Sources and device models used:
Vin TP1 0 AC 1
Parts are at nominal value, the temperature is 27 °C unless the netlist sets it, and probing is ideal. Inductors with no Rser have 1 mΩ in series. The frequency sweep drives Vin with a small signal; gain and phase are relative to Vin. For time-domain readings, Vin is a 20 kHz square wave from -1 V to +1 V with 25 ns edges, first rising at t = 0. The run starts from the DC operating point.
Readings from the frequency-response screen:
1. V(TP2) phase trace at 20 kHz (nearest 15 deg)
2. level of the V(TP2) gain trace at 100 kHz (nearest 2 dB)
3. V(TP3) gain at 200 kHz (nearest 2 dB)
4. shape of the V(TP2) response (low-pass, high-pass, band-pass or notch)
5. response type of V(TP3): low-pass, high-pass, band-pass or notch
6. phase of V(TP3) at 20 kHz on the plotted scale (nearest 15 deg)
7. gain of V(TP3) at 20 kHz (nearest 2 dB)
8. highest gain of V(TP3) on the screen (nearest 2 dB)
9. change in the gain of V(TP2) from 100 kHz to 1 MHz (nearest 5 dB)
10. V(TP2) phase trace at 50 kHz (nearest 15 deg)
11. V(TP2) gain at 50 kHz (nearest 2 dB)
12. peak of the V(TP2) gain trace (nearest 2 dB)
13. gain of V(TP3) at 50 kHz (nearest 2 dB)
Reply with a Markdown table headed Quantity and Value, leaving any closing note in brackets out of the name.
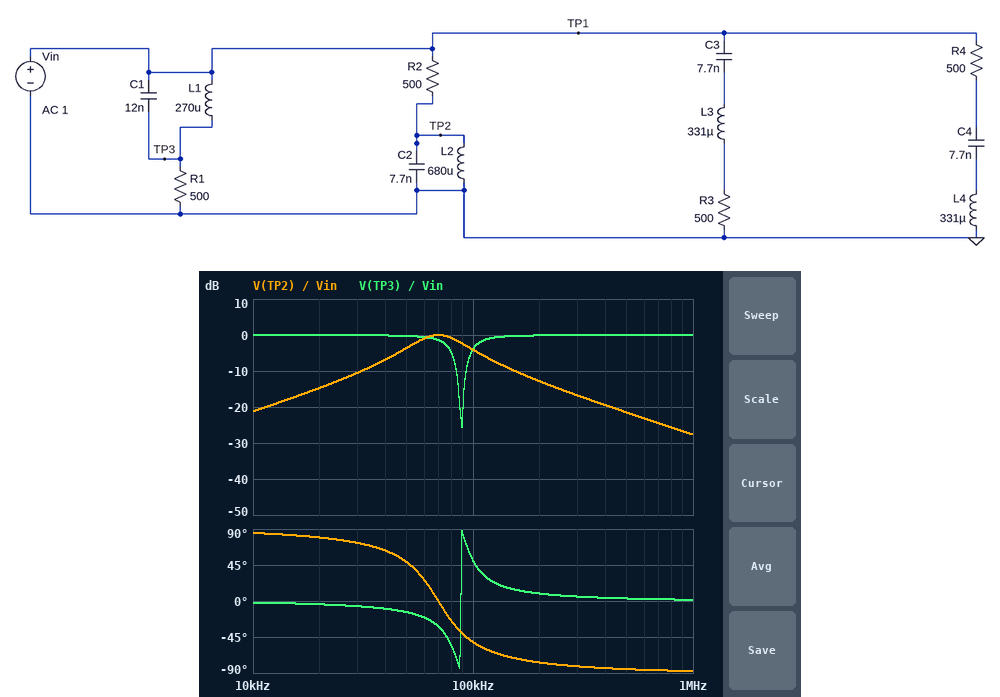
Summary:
| Quantity | Value |
|---|---|
| V(TP2) phase trace at 20 kHz | 75 deg |
| level of the V(TP2) gain trace at 100 kHz | -4 dB |
| V(TP3) gain at 200 kHz | 0 dB |
| shape of the V(TP2) response | band-pass |
| response type of V(TP3): low-pass, high-pass, band-pass or notch | notch |
| phase of V(TP3) at 20 kHz on the plotted scale | 0 deg |
| gain of V(TP3) at 20 kHz | 0 dB |
| highest gain of V(TP3) on the screen | 0 dB |
| change in the gain of V(TP2) from 100 kHz to 1 MHz | -25 dB |
| V(TP2) phase trace at 50 kHz | 45 deg |
| V(TP2) gain at 50 kHz | -4 dB |
| peak of the V(TP2) gain trace | 0 dB |
| gain of V(TP3) at 50 kHz | 0 dB |
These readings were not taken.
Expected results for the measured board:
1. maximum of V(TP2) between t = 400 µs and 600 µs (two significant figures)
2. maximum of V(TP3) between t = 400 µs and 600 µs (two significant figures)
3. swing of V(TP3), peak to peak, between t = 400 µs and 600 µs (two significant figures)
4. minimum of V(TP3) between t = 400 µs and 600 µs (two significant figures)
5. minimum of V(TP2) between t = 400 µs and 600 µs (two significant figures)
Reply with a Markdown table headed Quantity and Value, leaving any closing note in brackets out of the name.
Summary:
| Quantity | Value |
|---|---|
| maximum of V(TP2) between t = 400 µs and 600 µs | 830 mV |
| maximum of V(TP3) between t = 400 µs and 600 µs | 1.3 V |
| swing of V(TP3), peak to peak, between t = 400 µs and 600 µs | 2.6 V |
| minimum of V(TP3) between t = 400 µs and 600 µs | -1.3 V |
| minimum of V(TP2) between t = 400 µs and 600 µs | -830 mV |
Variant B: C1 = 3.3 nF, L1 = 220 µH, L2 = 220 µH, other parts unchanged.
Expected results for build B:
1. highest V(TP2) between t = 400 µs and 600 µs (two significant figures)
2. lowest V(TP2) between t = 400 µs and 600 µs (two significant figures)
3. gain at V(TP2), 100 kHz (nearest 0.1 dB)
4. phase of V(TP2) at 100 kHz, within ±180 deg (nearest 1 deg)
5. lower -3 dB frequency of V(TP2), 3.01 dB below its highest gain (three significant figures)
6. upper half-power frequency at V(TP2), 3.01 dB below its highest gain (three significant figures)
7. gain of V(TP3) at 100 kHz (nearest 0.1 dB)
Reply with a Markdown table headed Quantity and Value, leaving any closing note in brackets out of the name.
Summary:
| Quantity | Value |
|---|---|
| highest V(TP2) between t = 400 µs and 600 µs | 510 mV |
| lowest V(TP2) between t = 400 µs and 600 µs | -510 mV |
| gain at V(TP2), 100 kHz | -3.9 dB |
| phase of V(TP2) at 100 kHz, within ±180 deg | 50 deg |
| lower -3 dB frequency of V(TP2), 3.01 dB below its highest gain | 103 kHz |
| upper half-power frequency at V(TP2), 3.01 dB below its highest gain | 145 kHz |
| gain of V(TP3) at 100 kHz | -0.6 dB |
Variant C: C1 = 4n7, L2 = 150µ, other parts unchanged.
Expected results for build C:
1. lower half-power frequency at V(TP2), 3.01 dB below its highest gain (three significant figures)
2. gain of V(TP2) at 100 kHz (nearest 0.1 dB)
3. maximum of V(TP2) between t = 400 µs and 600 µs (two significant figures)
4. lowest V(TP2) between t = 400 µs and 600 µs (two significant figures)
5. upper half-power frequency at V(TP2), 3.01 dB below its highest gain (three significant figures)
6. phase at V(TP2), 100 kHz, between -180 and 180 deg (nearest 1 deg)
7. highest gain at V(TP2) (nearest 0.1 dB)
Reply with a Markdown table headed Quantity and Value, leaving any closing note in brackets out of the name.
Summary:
| Quantity | Value |
|---|---|
| lower half-power frequency at V(TP2), 3.01 dB below its highest gain | 129 kHz |
| gain of V(TP2) at 100 kHz | -9.7 dB |
| maximum of V(TP2) between t = 400 µs and 600 µs | 470 mV |
| lowest V(TP2) between t = 400 µs and 600 µs | -470 mV |
| upper half-power frequency at V(TP2), 3.01 dB below its highest gain | 170 kHz |
| phase at V(TP2), 100 kHz, between -180 and 180 deg | 71 deg |
| highest gain at V(TP2) | 0 dB |
